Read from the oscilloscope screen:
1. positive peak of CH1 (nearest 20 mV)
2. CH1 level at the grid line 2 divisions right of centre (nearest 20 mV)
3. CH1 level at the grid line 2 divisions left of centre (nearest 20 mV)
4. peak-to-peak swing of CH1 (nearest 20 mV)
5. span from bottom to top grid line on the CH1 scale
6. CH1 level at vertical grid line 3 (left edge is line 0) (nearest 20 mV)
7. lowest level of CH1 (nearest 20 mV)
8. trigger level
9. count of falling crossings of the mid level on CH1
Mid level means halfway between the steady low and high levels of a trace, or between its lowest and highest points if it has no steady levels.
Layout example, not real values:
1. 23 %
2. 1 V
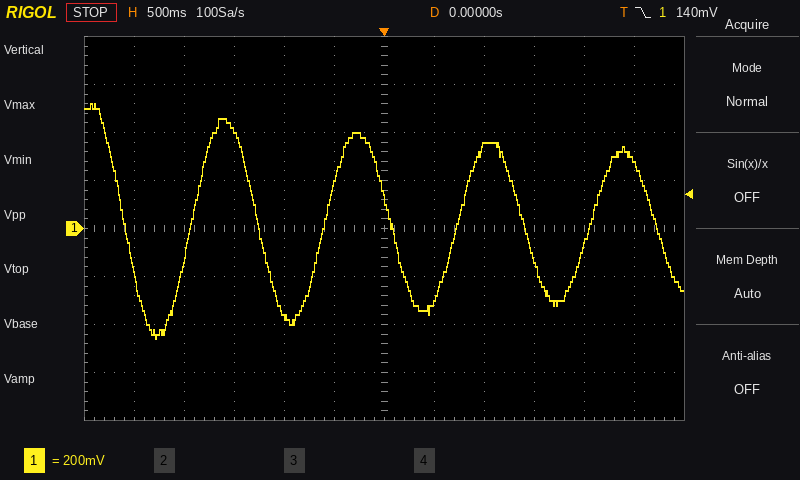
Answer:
1. 520 mV
2. 340 mV
3. -360 mV
4. 980 mV
5. 1.6 V
6. 400 mV
7. -460 mV
8. 140 mV
9. 5
